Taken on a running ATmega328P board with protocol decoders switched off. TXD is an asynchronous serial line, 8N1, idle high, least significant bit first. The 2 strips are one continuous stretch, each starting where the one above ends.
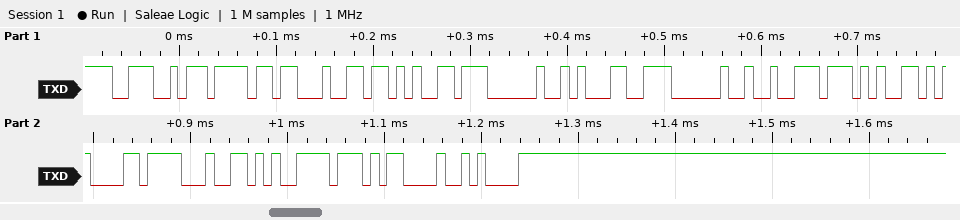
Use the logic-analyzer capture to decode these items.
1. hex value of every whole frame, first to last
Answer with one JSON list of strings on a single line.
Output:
["0x4E 0x6F 0x64 0x65 0x20 0x31 0x20 0x72 0x65 0x61 0x64 0x79 0x0D 0x0A"]
